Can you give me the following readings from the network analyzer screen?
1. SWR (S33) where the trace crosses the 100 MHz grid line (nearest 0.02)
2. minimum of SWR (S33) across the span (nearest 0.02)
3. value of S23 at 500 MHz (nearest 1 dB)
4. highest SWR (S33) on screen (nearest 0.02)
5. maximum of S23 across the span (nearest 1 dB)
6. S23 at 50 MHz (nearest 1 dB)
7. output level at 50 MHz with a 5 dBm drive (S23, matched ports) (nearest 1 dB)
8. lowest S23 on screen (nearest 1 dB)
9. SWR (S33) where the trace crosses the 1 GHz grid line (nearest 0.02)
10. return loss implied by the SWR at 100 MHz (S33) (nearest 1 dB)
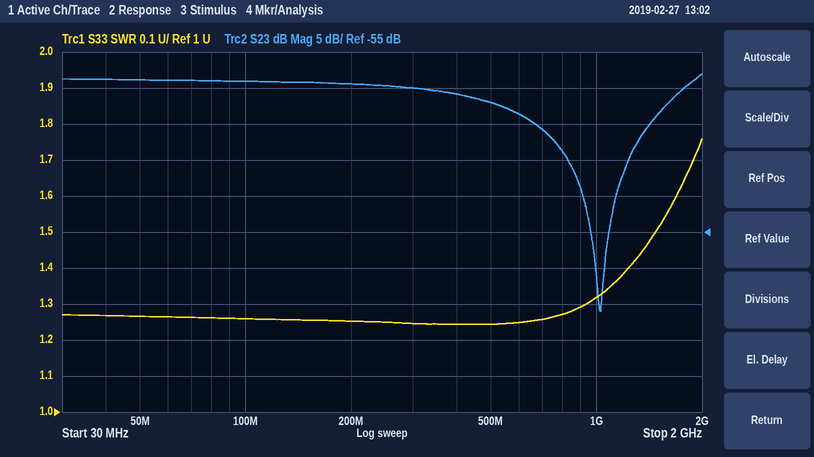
1.26
1.24
-37 dB
1.76
-33 dB
-34 dB
-29 dBm
-66 dB
1.32
19 dB
